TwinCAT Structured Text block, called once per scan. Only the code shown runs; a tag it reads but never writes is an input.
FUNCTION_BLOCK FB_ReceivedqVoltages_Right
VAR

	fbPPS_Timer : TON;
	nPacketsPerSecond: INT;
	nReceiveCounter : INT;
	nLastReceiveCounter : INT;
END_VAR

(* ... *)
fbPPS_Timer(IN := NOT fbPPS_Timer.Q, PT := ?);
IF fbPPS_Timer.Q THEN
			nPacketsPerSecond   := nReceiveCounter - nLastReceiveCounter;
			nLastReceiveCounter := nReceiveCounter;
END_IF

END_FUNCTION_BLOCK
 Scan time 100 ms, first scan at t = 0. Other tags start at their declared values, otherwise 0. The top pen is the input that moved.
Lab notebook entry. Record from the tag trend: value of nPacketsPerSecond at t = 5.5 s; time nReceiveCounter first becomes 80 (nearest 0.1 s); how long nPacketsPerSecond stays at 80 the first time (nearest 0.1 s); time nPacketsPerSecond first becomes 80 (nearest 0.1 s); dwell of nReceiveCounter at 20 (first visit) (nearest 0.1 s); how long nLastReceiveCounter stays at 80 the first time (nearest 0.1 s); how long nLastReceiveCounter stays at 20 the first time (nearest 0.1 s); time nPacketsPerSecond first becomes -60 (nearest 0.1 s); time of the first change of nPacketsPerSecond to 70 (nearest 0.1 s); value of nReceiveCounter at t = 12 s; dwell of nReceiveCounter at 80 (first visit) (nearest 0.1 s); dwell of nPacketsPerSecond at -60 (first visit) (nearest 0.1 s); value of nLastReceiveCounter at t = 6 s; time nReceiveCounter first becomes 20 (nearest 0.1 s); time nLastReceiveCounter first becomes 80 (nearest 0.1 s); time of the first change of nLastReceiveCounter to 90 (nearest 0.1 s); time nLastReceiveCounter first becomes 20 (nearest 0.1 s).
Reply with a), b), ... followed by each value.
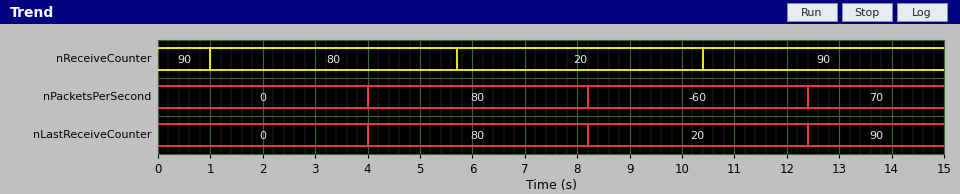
a) 80
b) 1.0 s
c) 4.2 s
d) 4.0 s
e) 4.7 s
f) 4.2 s
g) 4.2 s
h) 8.2 s
i) 12.4 s
j) 90
k) 4.7 s
l) 4.2 s
m) 80
n) 5.7 s
o) 4.0 s
p) 12.4 s
q) 8.2 s
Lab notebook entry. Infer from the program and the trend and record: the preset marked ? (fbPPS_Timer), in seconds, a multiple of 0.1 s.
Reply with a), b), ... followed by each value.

a) 4.0 s
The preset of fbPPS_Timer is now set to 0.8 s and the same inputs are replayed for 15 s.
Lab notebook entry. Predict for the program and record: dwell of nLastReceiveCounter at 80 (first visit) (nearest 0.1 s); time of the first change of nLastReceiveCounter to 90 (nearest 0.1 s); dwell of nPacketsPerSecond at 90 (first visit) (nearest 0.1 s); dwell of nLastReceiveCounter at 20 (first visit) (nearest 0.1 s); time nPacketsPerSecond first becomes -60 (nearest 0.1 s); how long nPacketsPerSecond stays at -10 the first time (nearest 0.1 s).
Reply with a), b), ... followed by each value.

a) 4.0 s
b) 0.8 s
c) 1.0 s
d) 5.0 s
e) 5.8 s
f) 1.0 s
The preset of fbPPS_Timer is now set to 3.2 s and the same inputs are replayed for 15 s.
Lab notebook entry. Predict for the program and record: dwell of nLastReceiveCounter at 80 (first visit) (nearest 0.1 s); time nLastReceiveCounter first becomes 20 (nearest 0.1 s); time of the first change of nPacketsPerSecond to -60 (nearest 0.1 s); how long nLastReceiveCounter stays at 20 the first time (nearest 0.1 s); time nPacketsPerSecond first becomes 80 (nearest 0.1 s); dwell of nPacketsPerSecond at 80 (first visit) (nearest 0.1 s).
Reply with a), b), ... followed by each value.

a) 3.4 s
b) 6.6 s
c) 6.6 s
d) 6.8 s
e) 3.2 s
f) 3.4 s
